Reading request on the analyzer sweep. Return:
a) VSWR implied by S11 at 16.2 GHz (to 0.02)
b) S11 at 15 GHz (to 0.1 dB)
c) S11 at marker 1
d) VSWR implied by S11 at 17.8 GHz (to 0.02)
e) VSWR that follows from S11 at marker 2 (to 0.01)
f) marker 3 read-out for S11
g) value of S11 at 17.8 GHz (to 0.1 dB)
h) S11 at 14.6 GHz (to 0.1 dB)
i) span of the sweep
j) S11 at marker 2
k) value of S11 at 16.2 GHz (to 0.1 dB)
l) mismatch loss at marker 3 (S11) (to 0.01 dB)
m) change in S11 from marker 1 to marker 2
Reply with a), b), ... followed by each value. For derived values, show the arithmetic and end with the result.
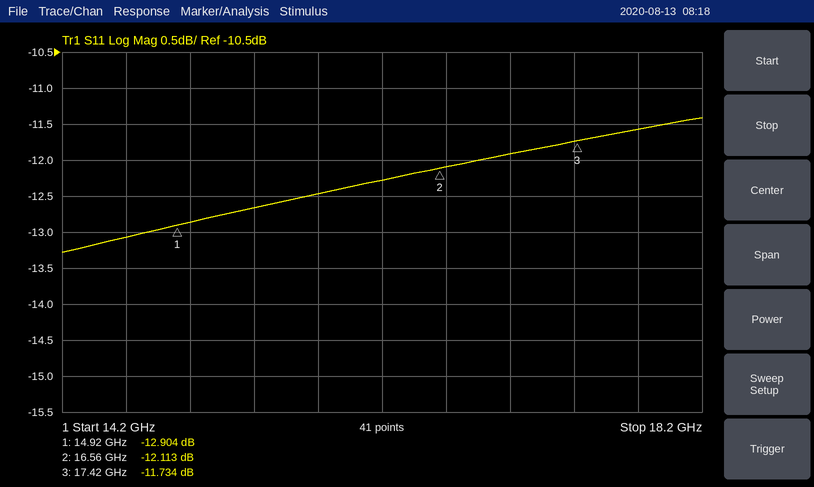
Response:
a) |Γ| = 10^(-12.3/20) = 0.2427; VSWR = (1 + 0.2427)/(1 − 0.2427) ≈ 1.64
b) -12.9 dB
c) -12.904 dB
d) |Γ| = 10^(-11.6/20) = 0.2630; VSWR = (1 + 0.2630)/(1 − 0.2630) ≈ 1.71, so 1.72 to the nearest 0.02
e) (1 + 0.2479)/(1 − 0.2479) ≈ 1.66
f) -11.734 dB
g) -11.6 dB
h) -13.1 dB
i) 4 GHz
j) -12.113 dB
k) -12.3 dB
l) −10 log10(1 − 10^(-11.734/10)) ≈ 0.30 dB
m) -12.113 − (-12.904) = 0.791 dB
